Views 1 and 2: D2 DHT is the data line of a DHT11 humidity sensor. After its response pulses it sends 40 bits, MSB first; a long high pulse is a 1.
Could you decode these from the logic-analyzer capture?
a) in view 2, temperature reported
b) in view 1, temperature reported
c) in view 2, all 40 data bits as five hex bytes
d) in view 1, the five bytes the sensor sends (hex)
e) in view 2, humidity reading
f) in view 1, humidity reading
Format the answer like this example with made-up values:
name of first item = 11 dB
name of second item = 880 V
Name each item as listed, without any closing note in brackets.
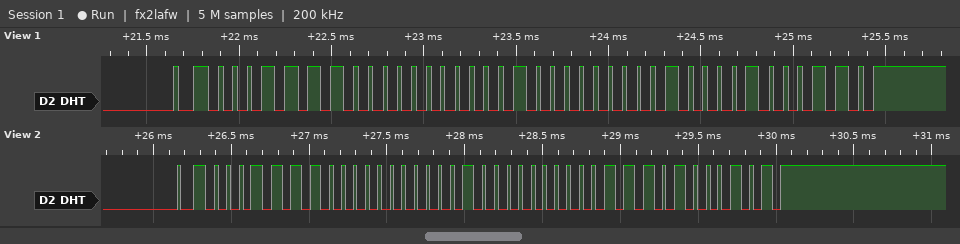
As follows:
in view 2, temperature reported = 32.7 °C
in view 1, temperature reported = 32.8 °C
in view 2, all 40 data bits as five hex bytes = 1E 00 20 07 45
in view 1, the five bytes the sensor sends = 1E 00 20 08 46
in view 2, humidity reading = 30 %
in view 1, humidity reading = 30 %
